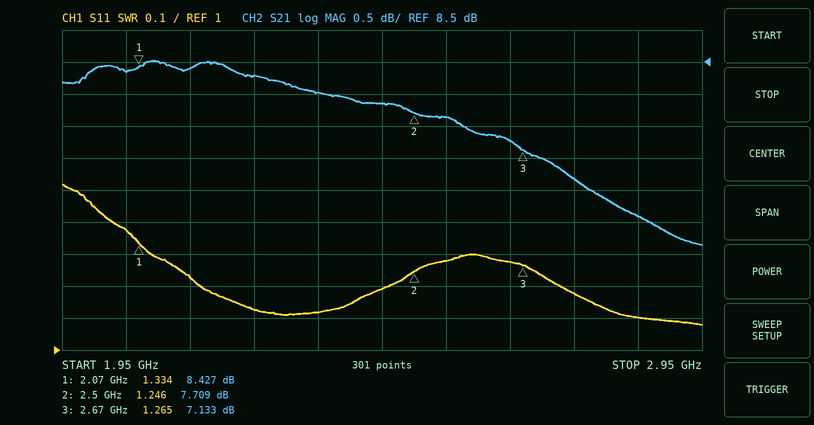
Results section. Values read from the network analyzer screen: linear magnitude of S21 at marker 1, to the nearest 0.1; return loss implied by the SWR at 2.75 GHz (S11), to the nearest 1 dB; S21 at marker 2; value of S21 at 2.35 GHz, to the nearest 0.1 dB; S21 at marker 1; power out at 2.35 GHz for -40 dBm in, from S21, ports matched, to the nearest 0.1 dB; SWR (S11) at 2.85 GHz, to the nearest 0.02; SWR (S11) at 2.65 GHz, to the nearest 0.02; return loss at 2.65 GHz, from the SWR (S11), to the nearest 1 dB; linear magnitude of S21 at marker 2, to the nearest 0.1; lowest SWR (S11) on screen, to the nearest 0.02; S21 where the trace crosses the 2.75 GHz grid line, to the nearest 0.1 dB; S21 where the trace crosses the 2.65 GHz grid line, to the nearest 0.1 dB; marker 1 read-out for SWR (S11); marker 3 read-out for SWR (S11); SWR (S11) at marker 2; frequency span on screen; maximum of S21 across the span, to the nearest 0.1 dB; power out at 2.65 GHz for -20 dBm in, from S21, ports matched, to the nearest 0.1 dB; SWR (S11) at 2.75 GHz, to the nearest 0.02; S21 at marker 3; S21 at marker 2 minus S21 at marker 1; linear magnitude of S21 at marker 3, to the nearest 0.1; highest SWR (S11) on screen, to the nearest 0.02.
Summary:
2.6
22 dB
7.709 dB
8.0 dB
8.427 dB
-32.0 dBm
1.10
1.28
18 dB
2.4
1.08
6.7 dB
7.3 dB
1.334
1.265
1.246
1 GHz
8.5 dB
-12.7 dBm
1.18
7.133 dB
-0.718 dB
2.3
1.52
